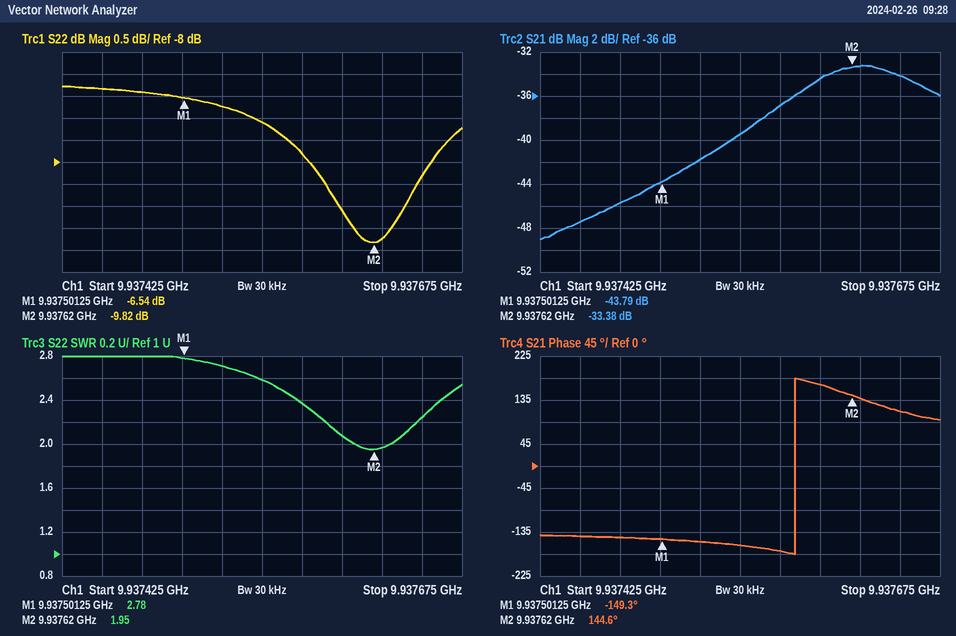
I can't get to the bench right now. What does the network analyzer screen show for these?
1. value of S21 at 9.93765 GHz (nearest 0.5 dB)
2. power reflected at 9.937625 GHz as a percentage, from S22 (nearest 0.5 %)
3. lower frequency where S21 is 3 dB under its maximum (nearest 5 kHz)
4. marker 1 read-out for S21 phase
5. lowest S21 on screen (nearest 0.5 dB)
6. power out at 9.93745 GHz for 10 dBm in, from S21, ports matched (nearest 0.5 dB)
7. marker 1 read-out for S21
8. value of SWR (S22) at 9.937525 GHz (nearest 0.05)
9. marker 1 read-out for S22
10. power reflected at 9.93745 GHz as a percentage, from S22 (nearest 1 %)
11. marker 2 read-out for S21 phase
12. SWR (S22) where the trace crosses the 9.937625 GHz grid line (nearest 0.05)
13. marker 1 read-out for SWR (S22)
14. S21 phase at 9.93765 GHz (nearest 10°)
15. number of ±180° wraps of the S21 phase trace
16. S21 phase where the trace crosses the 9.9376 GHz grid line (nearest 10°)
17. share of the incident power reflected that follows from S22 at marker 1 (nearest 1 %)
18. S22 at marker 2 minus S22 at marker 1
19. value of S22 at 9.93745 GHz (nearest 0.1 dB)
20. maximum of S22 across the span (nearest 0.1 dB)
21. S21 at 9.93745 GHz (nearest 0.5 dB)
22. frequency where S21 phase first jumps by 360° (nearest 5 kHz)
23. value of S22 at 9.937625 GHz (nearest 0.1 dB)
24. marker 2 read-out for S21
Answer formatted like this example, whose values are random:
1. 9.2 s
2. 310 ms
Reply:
1. -34.0 dB
2. 10.5 %
3. 9.937580 GHz
4. -149.3°
5. -49.0 dB
6. -37.5 dBm
7. -43.79 dB
8. 2.70
9. -6.54 dB
10. 23 %
11. 144.6°
12. 1.95
13. 2.78
14. 110°
15. 1
16. 170°
17. 22 %
18. -3.28 dB
19. -6.3 dB
20. -6.3 dB
21. -47.5 dB
22. 9.937585 GHz
23. -9.7 dB
24. -33.38 dB
